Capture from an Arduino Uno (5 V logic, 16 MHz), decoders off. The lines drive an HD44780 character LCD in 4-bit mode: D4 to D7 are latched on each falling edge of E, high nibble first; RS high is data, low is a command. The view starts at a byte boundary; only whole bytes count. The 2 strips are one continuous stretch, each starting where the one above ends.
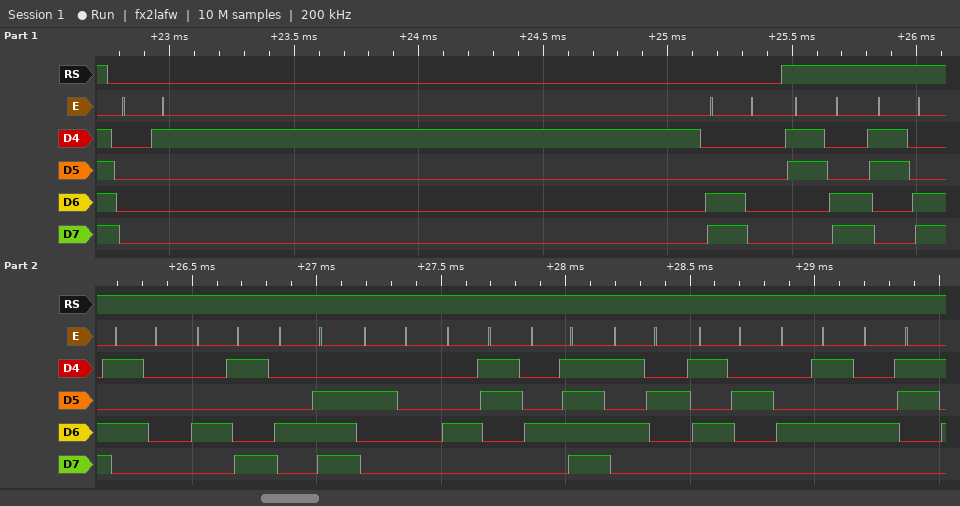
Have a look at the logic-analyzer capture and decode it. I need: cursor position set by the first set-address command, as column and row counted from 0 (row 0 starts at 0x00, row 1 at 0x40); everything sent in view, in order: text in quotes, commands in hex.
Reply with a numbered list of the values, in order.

1. column 0, row 1
2. 0x01 0xC0 "<<PIN CORREC"
